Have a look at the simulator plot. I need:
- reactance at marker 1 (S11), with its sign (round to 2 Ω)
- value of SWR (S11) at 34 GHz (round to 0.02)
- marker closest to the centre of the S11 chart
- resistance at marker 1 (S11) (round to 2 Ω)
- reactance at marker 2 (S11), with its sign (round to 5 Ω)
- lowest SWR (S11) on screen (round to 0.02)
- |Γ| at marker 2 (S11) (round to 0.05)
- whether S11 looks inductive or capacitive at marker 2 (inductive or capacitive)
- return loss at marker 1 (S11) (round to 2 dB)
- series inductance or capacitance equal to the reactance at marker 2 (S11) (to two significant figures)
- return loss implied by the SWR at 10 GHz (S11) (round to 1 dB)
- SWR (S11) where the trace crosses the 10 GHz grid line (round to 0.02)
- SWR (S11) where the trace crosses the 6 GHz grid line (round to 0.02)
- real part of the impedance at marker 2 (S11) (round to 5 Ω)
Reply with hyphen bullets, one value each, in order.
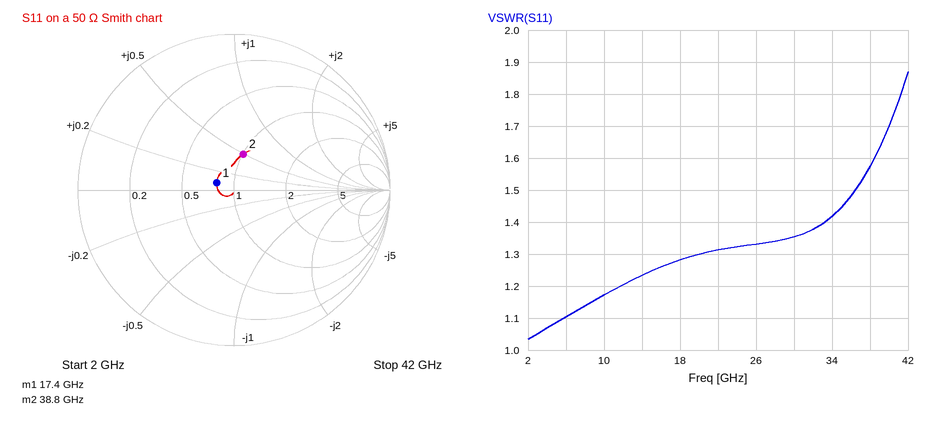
- +4 Ω
- 1.42
- marker 1
- 40 Ω
- +25 Ω
- 1.04
- 0.25
- inductive
- 18 dB
- 100 pH
- 22 dB
- 1.18
- 1.10
- 50 Ω
